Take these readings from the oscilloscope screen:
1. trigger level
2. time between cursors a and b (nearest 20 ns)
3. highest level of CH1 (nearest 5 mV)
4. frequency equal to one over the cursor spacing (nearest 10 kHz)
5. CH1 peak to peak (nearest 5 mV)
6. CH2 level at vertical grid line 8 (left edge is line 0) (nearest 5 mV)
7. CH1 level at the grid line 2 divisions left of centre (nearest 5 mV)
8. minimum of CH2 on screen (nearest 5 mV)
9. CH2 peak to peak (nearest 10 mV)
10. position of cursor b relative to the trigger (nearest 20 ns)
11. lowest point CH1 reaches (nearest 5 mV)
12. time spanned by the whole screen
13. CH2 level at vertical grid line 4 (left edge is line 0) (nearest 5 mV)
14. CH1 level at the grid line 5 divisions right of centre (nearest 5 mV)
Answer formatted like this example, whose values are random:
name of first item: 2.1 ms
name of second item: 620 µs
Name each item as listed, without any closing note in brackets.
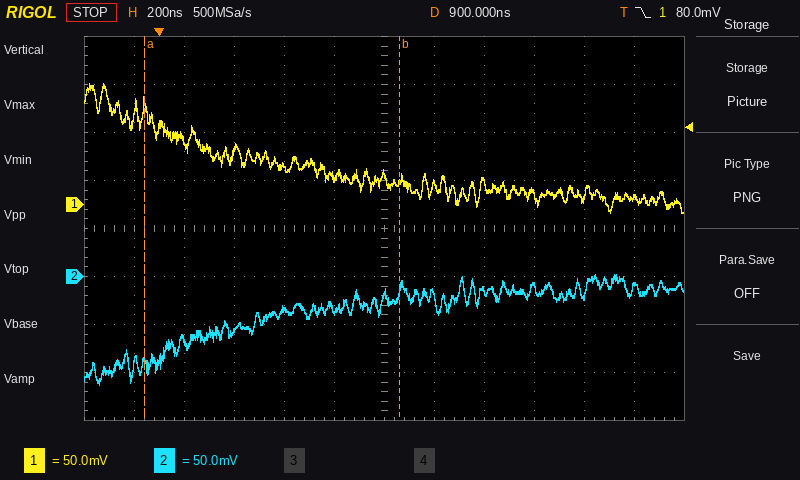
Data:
trigger level: 80.0 mV
time between cursors a and b: 1.02 µs
highest level of CH1: 125 mV
frequency equal to one over the cursor spacing: 980 kHz
CH1 peak to peak: 135 mV
CH2 level at vertical grid line 8 (left edge is line 0): -15 mV
CH1 level at the grid line 2 divisions left of centre: 40 mV
minimum of CH2 on screen: -110 mV
CH2 peak to peak: 110 mV
position of cursor b relative to the trigger: +960 ns
lowest point CH1 reaches: -10 mV
time spanned by the whole screen: 2.4 µs
CH2 level at vertical grid line 4 (left edge is line 0): -35 mV
CH1 level at the grid line 5 divisions right of centre: 5 mV
